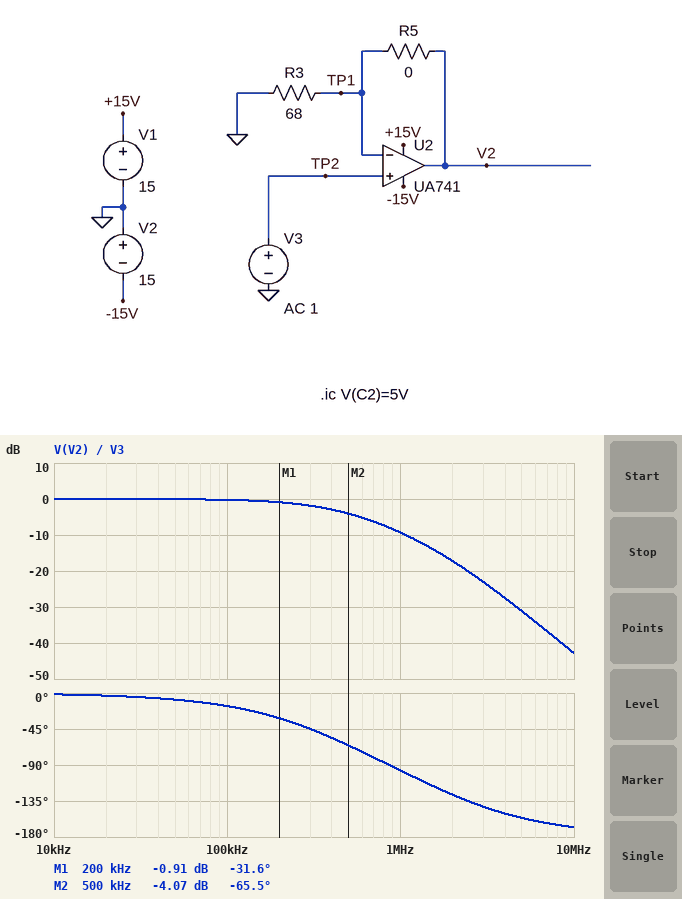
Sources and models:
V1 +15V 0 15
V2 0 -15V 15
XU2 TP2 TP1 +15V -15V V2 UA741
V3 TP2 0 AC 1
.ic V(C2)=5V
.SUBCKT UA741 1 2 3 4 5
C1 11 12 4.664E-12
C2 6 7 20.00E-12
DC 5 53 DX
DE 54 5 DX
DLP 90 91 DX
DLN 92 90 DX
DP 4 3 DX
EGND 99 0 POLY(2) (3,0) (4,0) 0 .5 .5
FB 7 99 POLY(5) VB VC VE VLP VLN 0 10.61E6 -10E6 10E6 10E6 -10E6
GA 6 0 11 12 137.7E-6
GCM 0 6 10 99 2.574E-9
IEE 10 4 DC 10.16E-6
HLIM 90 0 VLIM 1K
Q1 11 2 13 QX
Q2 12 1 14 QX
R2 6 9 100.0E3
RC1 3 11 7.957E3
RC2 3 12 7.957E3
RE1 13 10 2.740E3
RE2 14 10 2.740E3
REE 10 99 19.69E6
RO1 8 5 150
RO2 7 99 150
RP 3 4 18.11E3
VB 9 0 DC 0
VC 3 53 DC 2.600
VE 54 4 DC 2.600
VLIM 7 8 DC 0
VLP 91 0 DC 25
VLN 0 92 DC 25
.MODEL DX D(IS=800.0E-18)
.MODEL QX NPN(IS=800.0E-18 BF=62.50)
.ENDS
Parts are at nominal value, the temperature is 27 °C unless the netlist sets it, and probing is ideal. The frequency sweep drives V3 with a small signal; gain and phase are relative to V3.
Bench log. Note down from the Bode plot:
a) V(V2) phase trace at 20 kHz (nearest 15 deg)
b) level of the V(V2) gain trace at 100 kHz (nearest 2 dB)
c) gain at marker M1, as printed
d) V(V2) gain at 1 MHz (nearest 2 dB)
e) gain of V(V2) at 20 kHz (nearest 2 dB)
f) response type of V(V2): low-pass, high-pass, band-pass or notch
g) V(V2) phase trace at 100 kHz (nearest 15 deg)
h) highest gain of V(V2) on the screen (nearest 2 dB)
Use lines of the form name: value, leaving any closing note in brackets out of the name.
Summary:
V(V2) phase trace at 20 kHz: 0 deg
level of the V(V2) gain trace at 100 kHz: 0 dB
gain at marker M1, as printed: -0.91 dB
V(V2) gain at 1 MHz: -10 dB
gain of V(V2) at 20 kHz: 0 dB
response type of V(V2): low-pass, high-pass, band-pass or notch: low-pass
V(V2) phase trace at 100 kHz: -15 deg
highest gain of V(V2) on the screen: 0 dB
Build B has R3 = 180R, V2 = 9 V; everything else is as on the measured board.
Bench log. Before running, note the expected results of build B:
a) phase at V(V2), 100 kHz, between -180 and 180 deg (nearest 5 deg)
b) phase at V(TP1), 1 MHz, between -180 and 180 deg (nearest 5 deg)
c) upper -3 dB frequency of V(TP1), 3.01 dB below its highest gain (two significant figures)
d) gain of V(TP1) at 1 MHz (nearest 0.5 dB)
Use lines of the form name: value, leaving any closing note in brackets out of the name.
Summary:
phase at V(V2), 100 kHz, between -180 and 180 deg: -10 deg
phase at V(TP1), 1 MHz, between -180 and 180 deg: -85 deg
upper -3 dB frequency of V(TP1), 3.01 dB below its highest gain: 770 kHz
gain of V(TP1) at 1 MHz: -4.5 dB
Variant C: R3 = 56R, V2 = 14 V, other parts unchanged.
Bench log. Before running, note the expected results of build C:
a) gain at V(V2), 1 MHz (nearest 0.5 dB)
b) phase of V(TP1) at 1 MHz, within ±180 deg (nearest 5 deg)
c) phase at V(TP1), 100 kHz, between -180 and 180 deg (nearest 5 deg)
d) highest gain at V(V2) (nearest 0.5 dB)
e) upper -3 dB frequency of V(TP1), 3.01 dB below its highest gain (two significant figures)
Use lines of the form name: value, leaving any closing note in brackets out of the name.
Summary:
gain at V(V2), 1 MHz: -10.5 dB
phase of V(TP1) at 1 MHz, within ±180 deg: -100 deg
phase at V(TP1), 100 kHz, between -180 and 180 deg: -20 deg
highest gain at V(V2): 0 dB
upper -3 dB frequency of V(TP1), 3.01 dB below its highest gain: 340 kHz
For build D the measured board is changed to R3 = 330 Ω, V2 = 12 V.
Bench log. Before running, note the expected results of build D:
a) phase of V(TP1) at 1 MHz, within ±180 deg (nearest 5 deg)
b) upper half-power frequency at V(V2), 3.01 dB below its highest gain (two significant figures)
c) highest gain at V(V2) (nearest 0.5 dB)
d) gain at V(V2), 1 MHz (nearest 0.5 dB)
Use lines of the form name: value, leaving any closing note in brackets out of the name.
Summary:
phase of V(TP1) at 1 MHz, within ±180 deg: -75 deg
upper half-power frequency at V(V2), 3.01 dB below its highest gain: 1.0 MHz
highest gain at V(V2): 0 dB
gain at V(V2), 1 MHz: -3.0 dB
